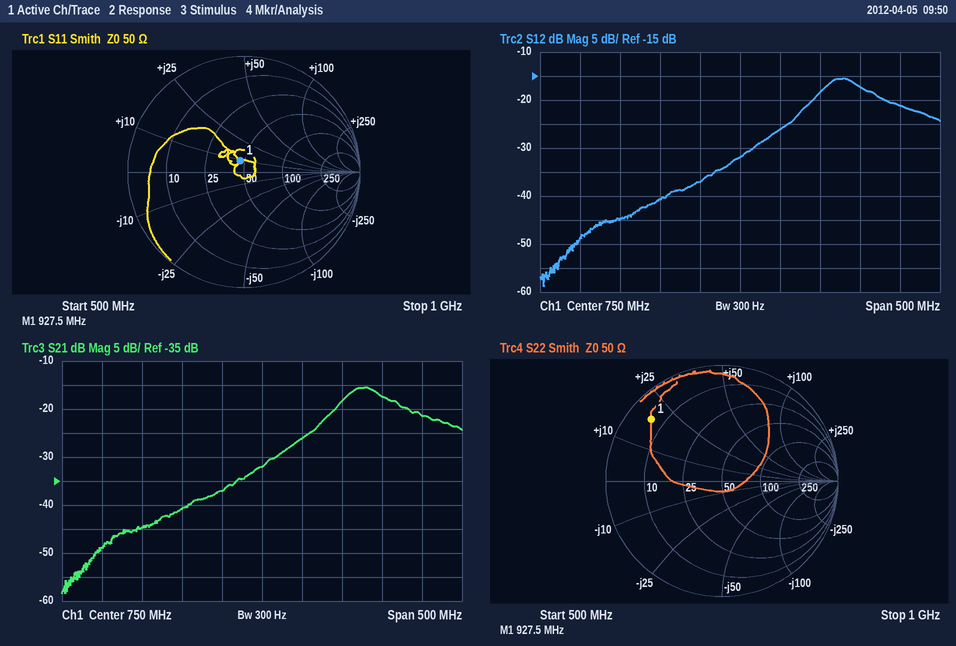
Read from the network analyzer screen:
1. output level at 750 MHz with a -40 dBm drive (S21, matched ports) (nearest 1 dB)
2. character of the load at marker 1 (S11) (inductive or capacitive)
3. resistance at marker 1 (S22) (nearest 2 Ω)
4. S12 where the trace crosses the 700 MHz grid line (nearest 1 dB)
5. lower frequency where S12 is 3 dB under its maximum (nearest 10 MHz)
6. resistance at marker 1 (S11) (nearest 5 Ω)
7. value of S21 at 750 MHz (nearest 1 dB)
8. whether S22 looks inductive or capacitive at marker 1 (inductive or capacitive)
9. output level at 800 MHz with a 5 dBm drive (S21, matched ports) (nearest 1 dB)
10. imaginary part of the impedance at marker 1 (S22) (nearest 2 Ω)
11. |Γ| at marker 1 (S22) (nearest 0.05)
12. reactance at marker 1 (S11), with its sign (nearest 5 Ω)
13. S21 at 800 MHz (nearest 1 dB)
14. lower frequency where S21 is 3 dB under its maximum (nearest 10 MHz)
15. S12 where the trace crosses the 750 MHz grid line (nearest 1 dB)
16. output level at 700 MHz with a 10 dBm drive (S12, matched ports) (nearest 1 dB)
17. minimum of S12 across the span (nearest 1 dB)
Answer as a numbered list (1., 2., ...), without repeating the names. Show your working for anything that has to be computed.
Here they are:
1. -40 dBm + (-32 dB) = -72 dBm
2. inductive
3. 6 Ω
4. -37 dB
5. 850 MHz
6. 45 Ω
7. -32 dB
8. inductive
9. 5 dBm + (-26 dB) = -21 dBm
10. +18 Ω
11. 0.80
12. +10 Ω
13. -26 dB
14. 850 MHz
15. -32 dB
16. 10 dBm + (-37 dB) = -27 dBm
17. -59 dB
